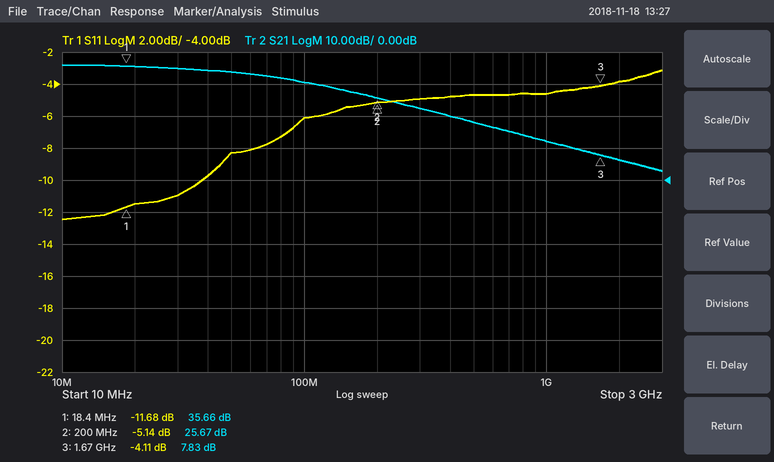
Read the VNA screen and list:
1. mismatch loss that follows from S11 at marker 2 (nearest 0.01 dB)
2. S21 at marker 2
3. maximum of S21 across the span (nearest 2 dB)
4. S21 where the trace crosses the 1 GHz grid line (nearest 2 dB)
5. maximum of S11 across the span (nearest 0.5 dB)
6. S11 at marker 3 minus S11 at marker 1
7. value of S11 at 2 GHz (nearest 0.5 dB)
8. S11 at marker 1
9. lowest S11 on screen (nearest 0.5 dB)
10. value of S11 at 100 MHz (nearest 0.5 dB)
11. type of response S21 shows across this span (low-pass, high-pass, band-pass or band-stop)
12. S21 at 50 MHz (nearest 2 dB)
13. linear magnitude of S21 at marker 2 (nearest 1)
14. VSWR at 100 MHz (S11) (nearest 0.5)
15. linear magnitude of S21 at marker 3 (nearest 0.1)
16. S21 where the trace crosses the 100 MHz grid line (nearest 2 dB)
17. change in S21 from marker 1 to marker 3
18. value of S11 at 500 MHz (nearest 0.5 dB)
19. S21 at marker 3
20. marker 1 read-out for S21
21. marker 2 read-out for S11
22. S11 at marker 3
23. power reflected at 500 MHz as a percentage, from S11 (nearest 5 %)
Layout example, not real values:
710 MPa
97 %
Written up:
1.59 dB
25.67 dB
36 dB
12 dB
-3.0 dB
7.57 dB
-4.0 dB
-11.68 dB
-12.5 dB
-6.0 dB
low-pass
34 dB
19
3.0
2.5
30 dB
-27.83 dB
-4.5 dB
7.83 dB
35.66 dB
-5.14 dB
-4.11 dB
35 %
